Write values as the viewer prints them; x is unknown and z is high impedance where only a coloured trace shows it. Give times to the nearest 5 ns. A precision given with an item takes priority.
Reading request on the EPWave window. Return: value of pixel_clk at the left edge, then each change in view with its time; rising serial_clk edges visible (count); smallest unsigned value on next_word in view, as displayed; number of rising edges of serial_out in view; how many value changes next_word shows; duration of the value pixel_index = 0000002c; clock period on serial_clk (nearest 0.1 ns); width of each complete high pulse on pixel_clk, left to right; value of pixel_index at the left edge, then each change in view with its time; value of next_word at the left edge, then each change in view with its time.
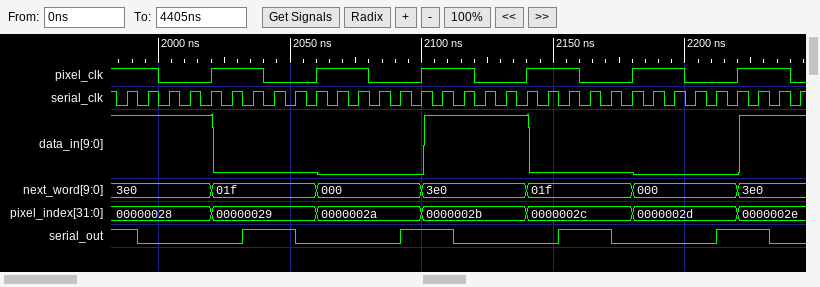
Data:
1, 0 at 2000 ns, 1 at 2020 ns, 0 at 2040 ns, 1 at 2060 ns, 0 at 2080 ns, 1 at 2100 ns, 0 at 2120 ns, 1 at 2140 ns, 0 at 2160 ns, 1 at 2180 ns, 0 at 2200 ns, 1 at 2220 ns, 0 at 2240 ns
33
000
4
6
40 ns
8 ns
20 ns, 20 ns, 20 ns, 20 ns, 20 ns, 20 ns
00000028, 00000029 at 2020 ns, 0000002a at 2060 ns, 0000002b at 2100 ns, 0000002c at 2140 ns, 0000002d at 2180 ns, 0000002e at 2220 ns
3e0, 01f at 2020 ns, 000 at 2060 ns, 3e0 at 2100 ns, 01f at 2140 ns, 000 at 2180 ns, 3e0 at 2220 ns
